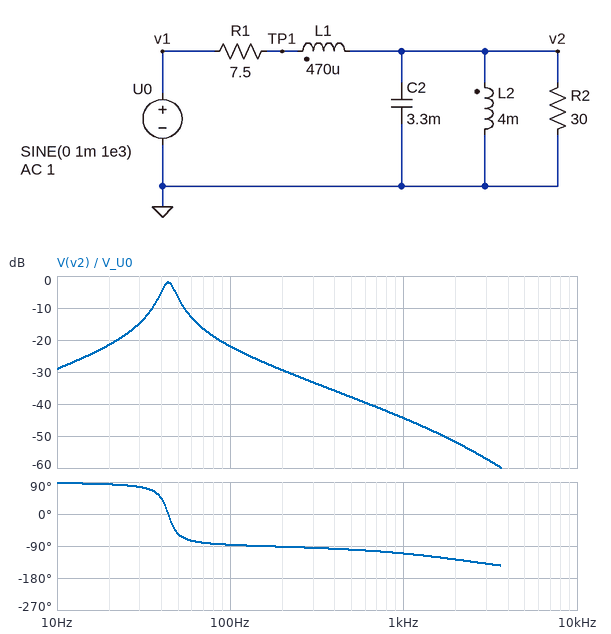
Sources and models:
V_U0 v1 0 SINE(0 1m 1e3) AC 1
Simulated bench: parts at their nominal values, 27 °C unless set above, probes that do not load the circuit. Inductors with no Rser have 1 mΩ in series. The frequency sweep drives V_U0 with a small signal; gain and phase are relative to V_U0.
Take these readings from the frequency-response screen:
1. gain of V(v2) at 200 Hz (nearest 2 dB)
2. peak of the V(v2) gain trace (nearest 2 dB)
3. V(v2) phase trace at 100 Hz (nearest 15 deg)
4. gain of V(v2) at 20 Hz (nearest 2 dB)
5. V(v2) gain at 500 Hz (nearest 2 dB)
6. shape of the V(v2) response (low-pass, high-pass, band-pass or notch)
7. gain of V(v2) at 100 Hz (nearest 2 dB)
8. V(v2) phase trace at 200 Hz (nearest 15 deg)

-30 dB
-2 dB
-90 deg
-22 dB
-38 dB
band-pass
-22 dB
-90 deg
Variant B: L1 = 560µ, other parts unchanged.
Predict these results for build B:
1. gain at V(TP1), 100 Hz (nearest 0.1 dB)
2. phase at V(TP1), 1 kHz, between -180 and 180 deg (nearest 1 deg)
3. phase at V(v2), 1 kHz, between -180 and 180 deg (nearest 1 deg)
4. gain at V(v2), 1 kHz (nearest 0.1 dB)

-29.7 dB
65 deg
-115 deg
-44.7 dB
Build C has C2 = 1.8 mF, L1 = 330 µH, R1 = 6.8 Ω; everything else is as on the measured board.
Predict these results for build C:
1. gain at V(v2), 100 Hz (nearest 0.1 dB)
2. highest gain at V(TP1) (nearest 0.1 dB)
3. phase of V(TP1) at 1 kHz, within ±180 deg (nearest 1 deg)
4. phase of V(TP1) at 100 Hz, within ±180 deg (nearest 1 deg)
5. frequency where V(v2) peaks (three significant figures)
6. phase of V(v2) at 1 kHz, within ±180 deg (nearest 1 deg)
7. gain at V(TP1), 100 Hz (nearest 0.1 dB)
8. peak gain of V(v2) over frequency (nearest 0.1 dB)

-14.2 dB
0 dB
74 deg
-77 deg
59.4 Hz
-106 deg
-15.6 dB
-1.8 dB
